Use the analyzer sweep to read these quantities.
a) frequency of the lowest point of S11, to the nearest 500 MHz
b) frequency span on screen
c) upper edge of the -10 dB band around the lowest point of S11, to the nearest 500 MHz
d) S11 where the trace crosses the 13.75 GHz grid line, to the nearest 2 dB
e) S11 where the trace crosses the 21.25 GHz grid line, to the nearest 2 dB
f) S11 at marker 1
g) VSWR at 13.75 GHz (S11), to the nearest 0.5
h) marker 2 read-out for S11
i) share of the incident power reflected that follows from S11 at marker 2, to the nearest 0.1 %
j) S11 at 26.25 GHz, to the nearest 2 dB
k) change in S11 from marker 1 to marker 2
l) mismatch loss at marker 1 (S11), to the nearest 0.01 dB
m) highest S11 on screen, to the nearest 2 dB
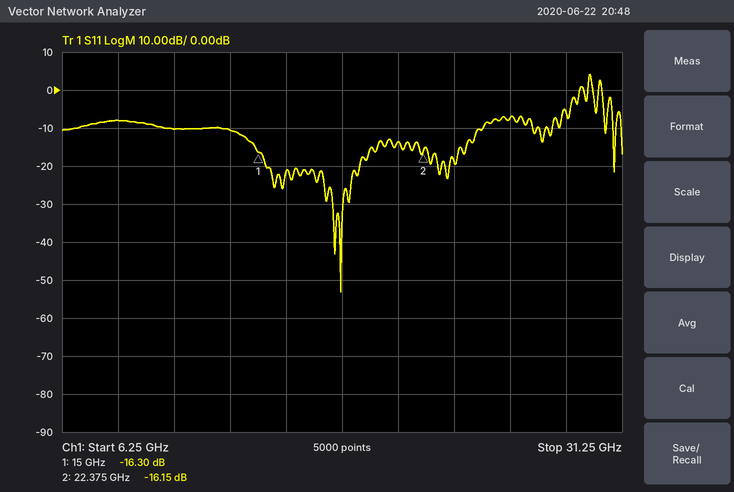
18.5 GHz
25 GHz
25.0 GHz
-10 dB
-14 dB
-16.30 dB
2.0
-16.15 dB
2.4 %
-8 dB
0.15 dB
0.10 dB
4 dB
